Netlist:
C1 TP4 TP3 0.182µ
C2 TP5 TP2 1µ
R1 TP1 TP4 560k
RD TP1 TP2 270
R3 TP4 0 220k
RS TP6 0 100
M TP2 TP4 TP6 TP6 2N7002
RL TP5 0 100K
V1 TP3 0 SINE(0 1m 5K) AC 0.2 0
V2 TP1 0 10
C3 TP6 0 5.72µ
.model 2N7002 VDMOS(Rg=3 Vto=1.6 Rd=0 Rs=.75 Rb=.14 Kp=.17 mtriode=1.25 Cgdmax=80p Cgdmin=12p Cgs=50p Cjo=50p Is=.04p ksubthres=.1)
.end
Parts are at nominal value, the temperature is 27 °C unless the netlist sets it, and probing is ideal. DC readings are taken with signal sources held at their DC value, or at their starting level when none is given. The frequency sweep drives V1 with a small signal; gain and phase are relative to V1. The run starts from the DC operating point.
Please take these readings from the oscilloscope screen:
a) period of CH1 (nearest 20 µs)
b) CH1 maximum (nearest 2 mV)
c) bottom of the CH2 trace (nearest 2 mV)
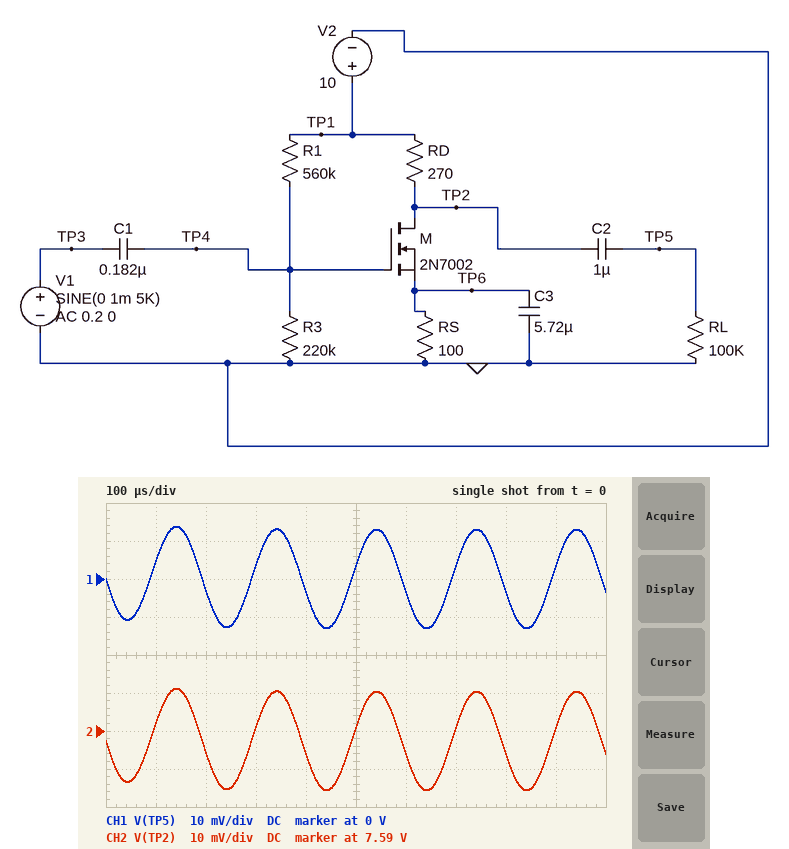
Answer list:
200 µs
14 mV
7.574 V
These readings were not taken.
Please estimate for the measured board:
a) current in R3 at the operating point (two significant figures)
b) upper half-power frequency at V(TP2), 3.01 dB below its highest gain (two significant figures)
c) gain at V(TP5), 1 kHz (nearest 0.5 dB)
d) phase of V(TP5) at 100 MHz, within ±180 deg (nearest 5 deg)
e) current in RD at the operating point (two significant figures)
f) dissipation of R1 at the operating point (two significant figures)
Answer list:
13 µA
16 MHz
17.0 dB
80 deg
8.9 mA
92 µW
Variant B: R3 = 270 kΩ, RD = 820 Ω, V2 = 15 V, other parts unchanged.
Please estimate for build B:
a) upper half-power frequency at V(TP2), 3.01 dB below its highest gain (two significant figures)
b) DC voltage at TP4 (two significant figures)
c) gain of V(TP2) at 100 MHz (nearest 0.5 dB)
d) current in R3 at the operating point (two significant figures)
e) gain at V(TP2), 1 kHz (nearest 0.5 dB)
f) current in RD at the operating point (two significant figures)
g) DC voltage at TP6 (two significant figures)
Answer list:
1.5 GHz
4.9 V
-14.5 dB
18 µA
-30.5 dB
16 mA
1.6 V
